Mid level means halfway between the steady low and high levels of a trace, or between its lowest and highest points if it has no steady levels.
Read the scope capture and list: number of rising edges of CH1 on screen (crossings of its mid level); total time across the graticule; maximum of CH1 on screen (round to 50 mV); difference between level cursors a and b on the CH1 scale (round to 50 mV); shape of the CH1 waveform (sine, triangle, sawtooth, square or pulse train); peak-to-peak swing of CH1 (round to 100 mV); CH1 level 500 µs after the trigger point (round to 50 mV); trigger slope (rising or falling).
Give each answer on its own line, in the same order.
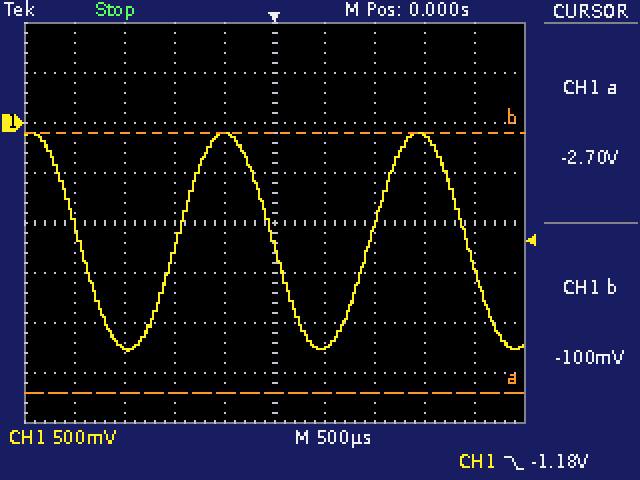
2
5 ms
-100 mV
2.60 V
sine
2.20 V
-2.25 V
falling
